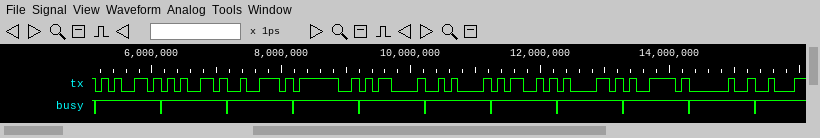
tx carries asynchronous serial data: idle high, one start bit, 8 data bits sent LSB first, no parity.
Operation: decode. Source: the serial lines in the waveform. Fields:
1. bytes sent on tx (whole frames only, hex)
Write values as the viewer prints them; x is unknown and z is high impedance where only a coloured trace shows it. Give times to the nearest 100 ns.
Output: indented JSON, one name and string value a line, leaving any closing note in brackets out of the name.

{
  "bytes sent on tx": "65, 65, 72, 3F, 0D, 0A, 4D, 61, 79, 20"
}
